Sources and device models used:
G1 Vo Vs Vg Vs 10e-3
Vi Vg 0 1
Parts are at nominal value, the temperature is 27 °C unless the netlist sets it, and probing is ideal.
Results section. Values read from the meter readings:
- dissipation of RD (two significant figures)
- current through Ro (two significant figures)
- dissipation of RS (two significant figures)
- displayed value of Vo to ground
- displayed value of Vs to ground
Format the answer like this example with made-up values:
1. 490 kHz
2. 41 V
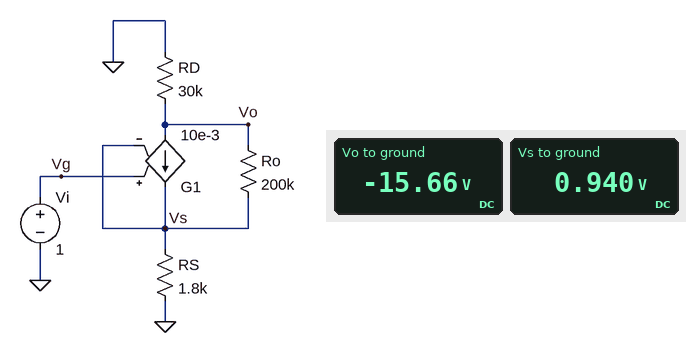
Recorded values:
1. 8.2 mW
2. 83 µA
3. 490 µW
4. -15.66 V
5. 0.940 V
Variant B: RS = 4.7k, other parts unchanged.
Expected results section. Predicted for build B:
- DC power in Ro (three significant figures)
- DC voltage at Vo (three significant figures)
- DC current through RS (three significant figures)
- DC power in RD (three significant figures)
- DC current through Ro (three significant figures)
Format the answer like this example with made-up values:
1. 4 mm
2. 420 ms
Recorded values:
1. 259 µW
2. -6.23 V
3. 208 µA
4. 1.29 mW
5. 36.0 µA
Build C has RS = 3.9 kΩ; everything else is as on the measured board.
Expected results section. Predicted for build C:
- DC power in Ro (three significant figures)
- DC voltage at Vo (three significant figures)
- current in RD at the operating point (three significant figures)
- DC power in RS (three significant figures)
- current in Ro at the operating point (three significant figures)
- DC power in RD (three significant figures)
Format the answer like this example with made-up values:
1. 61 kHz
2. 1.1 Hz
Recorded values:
1. 356 µW
2. -7.47 V
3. 249 µA
4. 242 µW
5. 42.2 µA
6. 1.86 mW
